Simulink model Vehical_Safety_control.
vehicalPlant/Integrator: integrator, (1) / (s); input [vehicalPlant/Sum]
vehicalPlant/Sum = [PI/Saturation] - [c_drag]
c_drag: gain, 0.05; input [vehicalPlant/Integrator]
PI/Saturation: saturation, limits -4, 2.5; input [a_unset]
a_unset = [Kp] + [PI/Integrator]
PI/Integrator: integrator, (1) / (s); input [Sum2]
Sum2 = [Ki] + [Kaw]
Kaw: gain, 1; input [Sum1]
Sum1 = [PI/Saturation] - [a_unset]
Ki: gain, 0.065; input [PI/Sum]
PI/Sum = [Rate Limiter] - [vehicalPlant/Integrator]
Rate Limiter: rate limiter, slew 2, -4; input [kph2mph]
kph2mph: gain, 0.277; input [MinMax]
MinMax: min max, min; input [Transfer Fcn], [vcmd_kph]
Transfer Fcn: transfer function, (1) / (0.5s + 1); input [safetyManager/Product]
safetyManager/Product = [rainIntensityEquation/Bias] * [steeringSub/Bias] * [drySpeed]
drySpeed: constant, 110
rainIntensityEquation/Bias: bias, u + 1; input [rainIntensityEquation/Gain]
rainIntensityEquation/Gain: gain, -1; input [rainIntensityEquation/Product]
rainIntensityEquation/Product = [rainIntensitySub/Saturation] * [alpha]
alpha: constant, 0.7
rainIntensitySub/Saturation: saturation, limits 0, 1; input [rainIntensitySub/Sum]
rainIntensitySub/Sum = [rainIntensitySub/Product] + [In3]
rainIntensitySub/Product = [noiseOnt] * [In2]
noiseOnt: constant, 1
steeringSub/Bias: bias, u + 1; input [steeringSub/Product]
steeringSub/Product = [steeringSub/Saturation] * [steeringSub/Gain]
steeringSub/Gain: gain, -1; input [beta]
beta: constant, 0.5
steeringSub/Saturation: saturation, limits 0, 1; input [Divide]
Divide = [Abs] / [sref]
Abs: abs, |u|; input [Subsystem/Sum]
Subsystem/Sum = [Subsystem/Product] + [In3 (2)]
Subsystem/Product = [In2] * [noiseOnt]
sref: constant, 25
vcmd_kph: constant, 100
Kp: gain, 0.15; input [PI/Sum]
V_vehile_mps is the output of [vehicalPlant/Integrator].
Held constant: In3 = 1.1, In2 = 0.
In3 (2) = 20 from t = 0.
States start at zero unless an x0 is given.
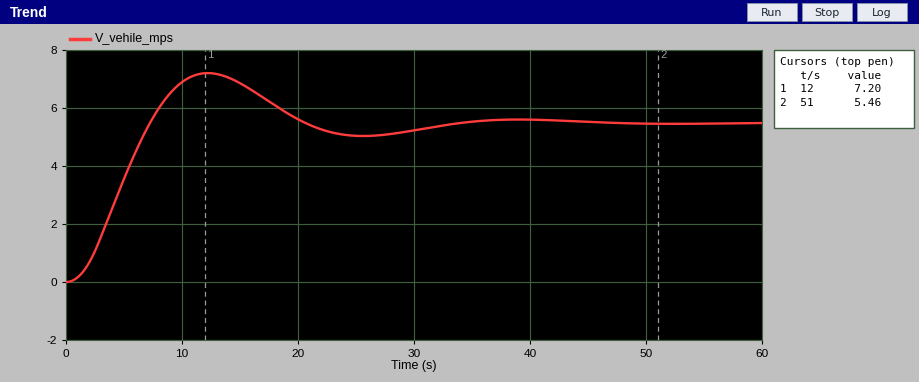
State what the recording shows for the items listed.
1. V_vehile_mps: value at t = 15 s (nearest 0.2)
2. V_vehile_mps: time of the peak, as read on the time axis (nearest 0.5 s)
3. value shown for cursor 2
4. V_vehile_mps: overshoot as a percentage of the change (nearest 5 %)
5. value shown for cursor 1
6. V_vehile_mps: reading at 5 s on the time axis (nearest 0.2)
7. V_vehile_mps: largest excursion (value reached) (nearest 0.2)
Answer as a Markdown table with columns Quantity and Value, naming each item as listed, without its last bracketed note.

| Quantity | Value |
|---|---|
| V_vehile_mps: value at t = 15 s | 6.8 |
| V_vehile_mps: time of the peak, as read on the time axis | 12.0 s |
| value shown for cursor 2 | 5.46 |
| V_vehile_mps: overshoot as a percentage of the change | 30 % |
| value shown for cursor 1 | 7.20 |
| V_vehile_mps: reading at 5 s on the time axis | 3.6 |
| V_vehile_mps: largest excursion (value reached) | 7.2 |
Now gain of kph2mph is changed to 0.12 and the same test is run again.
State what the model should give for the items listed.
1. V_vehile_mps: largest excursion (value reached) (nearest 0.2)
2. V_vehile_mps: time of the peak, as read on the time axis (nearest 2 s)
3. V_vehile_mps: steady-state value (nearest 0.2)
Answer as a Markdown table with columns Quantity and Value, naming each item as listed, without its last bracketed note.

| Quantity | Value |
|---|---|
| V_vehile_mps: largest excursion (value reached) | 3.2 |
| V_vehile_mps: time of the peak, as read on the time axis | 12 s |
| V_vehile_mps: steady-state value | 2.4 |
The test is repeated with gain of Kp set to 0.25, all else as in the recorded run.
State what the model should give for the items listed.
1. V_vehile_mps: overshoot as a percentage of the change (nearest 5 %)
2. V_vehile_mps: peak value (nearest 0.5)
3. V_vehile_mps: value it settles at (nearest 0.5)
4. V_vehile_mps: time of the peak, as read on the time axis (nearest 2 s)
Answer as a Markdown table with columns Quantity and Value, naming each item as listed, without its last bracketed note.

| Quantity | Value |
|---|---|
| V_vehile_mps: overshoot as a percentage of the change | 20 % |
| V_vehile_mps: peak value | 6.5 |
| V_vehile_mps: value it settles at | 5.5 |
| V_vehile_mps: time of the peak, as read on the time axis | 12 s |
